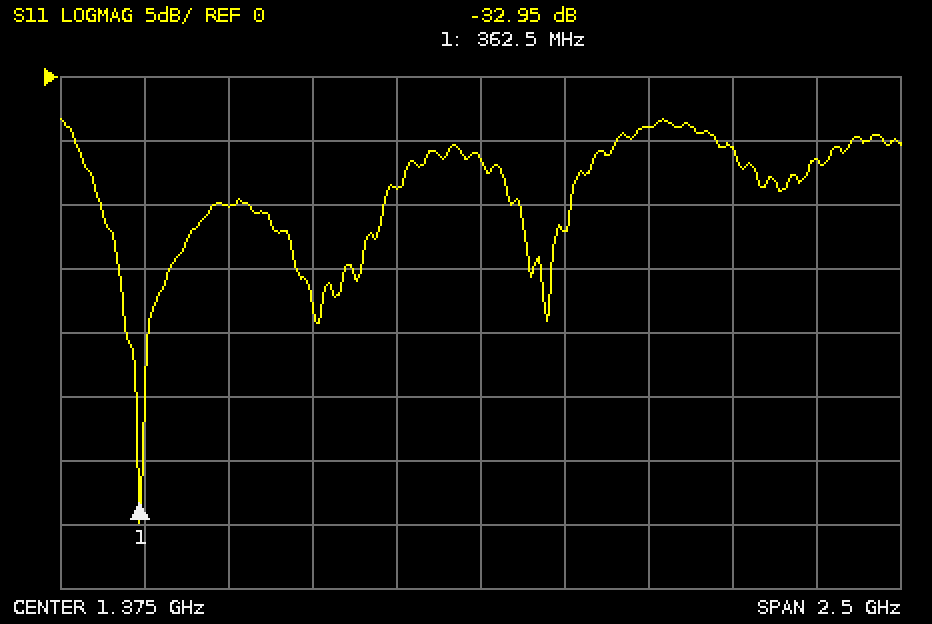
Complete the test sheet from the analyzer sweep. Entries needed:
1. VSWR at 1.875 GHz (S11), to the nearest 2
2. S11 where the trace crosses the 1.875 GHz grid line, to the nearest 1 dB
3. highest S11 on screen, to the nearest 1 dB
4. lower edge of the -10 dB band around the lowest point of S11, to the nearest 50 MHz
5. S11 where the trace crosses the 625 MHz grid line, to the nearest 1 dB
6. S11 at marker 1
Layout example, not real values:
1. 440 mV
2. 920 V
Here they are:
1. 4
2. -4 dB
3. -3 dB
4. 250 MHz
5. -10 dB
6. -32.95 dB
